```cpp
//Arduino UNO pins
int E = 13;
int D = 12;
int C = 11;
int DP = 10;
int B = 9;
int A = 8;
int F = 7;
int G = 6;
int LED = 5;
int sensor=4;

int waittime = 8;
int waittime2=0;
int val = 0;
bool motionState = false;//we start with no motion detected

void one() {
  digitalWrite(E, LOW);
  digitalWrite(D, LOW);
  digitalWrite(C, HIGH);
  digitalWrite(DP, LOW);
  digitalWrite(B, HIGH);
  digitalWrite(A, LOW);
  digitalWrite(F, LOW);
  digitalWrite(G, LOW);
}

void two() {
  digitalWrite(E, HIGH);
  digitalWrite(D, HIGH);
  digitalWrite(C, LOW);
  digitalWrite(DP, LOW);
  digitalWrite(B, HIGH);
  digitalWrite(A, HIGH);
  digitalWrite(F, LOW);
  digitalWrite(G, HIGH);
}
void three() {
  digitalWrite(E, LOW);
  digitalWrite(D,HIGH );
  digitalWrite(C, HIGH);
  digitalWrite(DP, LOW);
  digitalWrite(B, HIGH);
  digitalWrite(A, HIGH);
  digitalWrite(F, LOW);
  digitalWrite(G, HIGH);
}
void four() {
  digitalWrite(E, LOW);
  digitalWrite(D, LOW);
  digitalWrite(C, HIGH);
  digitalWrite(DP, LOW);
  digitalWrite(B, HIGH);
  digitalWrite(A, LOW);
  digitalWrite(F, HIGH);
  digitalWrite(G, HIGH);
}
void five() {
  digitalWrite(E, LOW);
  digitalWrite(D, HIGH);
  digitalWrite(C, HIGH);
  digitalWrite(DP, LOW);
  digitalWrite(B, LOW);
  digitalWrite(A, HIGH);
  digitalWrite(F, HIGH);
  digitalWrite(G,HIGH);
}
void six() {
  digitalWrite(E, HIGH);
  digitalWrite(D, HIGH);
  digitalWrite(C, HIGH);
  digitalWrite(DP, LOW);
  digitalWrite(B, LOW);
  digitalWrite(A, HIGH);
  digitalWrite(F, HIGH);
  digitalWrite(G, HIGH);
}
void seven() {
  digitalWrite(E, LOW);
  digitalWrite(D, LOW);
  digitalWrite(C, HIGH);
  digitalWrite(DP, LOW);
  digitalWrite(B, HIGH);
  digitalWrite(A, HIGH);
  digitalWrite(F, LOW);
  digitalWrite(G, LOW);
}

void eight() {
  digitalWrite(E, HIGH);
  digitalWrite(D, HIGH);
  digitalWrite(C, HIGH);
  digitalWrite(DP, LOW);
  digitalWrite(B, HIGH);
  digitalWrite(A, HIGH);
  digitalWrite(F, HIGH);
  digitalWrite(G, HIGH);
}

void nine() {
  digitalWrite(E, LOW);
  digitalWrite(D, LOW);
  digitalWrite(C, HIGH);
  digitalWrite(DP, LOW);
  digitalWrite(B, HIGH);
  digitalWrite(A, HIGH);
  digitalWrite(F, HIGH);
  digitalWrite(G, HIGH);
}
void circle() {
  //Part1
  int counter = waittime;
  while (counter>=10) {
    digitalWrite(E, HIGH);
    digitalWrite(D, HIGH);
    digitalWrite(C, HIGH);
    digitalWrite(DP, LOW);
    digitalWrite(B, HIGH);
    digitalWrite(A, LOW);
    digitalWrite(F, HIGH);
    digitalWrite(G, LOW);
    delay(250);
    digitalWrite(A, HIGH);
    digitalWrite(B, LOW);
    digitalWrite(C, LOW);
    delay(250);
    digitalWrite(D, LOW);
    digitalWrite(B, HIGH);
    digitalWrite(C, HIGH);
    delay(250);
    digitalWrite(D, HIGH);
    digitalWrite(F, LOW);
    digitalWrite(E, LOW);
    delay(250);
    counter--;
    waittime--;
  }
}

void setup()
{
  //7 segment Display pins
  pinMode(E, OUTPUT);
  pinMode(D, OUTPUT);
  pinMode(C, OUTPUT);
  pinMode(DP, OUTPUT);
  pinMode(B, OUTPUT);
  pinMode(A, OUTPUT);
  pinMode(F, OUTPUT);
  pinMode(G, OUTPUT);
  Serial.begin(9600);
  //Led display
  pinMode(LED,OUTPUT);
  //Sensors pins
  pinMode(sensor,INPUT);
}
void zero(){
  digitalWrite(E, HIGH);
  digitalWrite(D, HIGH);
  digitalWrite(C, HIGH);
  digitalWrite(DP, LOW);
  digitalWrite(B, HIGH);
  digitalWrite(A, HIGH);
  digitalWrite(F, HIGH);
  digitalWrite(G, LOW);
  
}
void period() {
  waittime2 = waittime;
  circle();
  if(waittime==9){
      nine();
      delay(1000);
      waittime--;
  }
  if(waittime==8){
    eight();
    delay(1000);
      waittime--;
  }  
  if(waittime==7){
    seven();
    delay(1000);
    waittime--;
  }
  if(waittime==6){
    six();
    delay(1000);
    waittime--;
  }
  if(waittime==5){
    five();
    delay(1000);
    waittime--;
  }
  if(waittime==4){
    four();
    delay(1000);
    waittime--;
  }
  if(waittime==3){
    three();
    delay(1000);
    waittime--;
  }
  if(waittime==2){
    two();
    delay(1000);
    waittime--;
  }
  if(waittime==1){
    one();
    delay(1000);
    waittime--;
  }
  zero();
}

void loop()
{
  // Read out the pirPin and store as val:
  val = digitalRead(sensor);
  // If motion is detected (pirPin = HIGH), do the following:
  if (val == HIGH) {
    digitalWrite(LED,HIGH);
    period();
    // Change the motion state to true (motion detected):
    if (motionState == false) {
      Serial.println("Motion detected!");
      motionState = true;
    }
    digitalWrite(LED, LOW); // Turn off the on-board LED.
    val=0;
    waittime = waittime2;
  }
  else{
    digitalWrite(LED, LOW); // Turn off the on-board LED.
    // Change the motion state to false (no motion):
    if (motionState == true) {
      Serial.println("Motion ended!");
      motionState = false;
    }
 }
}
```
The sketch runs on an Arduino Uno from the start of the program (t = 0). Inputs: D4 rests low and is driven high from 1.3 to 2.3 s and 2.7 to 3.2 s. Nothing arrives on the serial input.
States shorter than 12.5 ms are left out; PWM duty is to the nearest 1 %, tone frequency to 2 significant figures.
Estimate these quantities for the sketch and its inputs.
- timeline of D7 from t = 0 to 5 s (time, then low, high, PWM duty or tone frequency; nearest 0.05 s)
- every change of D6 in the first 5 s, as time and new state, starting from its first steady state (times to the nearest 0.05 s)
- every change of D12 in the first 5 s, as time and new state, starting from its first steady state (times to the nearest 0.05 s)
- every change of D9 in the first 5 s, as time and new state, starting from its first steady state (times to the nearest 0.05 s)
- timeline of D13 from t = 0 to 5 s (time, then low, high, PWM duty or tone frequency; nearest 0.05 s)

0 s low; 1.3 s high; 2.3 s low; 3.3 s high
0 s low; 1.3 s high; 2.3 s low; 3.3 s high
0 s low; 1.3 s high; 2.3 s low; 3.3 s high
0 s low; 1.3 s high; 3.3 s low
0 s low; 1.3 s high; 2.3 s low; 3.3 s high; 4.3 s low
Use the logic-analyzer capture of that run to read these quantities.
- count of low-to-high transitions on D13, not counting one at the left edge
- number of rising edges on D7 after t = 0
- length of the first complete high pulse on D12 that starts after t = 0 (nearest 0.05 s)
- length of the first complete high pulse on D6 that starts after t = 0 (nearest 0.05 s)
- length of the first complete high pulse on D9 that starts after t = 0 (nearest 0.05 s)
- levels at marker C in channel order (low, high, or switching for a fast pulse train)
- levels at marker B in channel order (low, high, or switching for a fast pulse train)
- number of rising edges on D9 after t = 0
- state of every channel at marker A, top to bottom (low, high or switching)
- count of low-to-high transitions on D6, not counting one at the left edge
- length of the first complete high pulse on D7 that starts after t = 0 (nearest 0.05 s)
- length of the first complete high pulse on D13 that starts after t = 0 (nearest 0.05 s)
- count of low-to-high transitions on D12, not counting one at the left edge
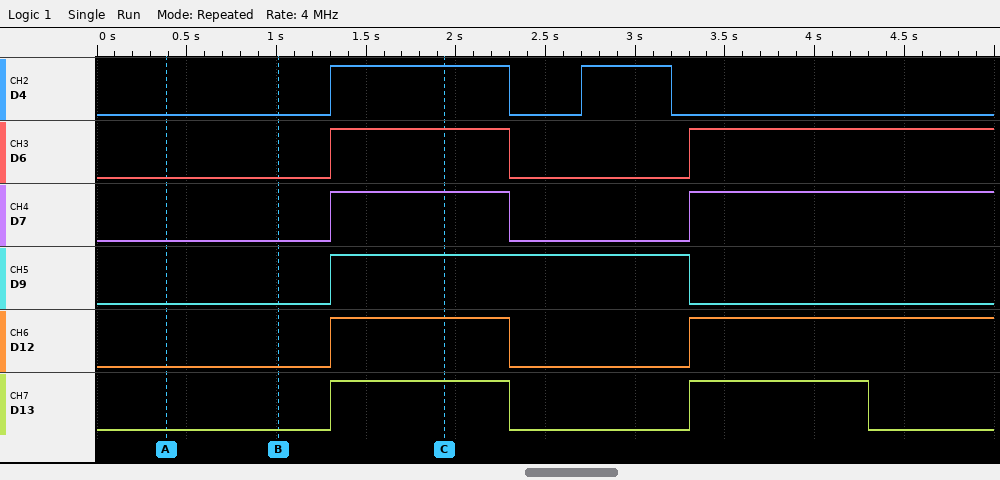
2
2
1.00 s
1.00 s
2.00 s
D4 high, D6 high, D7 high, D9 high, D12 high, D13 high
D4 low, D6 low, D7 low, D9 low, D12 low, D13 low
1
D4 low, D6 low, D7 low, D9 low, D12 low, D13 low
2
1.00 s
1.00 s
2
